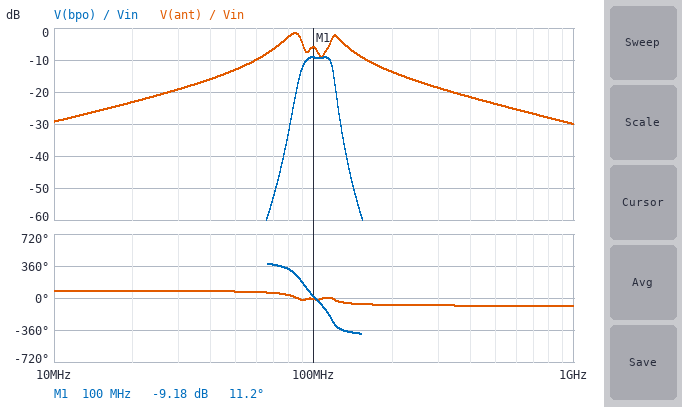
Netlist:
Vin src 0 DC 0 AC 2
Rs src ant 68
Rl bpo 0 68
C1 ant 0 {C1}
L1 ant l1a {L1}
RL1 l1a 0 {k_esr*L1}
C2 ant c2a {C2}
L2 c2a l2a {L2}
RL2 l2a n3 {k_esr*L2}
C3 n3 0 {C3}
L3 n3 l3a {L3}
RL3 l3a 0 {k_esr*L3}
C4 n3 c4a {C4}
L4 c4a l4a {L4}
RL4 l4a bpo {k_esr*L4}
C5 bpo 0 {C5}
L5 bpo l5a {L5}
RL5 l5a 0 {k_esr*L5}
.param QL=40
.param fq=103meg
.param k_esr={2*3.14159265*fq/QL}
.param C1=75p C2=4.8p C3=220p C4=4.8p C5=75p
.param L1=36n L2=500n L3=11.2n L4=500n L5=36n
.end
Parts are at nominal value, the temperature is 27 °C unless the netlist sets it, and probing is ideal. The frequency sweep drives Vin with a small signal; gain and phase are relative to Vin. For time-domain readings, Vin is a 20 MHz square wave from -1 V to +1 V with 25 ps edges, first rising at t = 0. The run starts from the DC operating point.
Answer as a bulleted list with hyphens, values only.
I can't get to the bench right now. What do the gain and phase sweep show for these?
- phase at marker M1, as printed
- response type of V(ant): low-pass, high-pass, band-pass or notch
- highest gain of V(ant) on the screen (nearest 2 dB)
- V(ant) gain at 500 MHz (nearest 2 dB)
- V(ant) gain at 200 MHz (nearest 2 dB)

- 11.2 deg
- band-pass
- -2 dB
- -24 dB
- -14 dB
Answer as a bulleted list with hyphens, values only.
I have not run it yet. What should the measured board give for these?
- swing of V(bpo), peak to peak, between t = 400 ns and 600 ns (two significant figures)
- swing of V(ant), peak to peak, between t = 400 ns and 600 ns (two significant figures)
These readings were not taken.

- 180 mV
- 890 mV
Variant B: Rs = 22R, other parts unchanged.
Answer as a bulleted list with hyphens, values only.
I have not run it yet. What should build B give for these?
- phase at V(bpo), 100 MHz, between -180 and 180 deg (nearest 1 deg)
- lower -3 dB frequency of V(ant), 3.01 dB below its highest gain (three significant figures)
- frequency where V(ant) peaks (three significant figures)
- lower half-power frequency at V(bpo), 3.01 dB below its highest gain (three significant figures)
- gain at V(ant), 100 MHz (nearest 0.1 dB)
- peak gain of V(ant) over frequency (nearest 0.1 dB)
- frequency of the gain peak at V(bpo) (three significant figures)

- 18 deg
- 57.3 MHz
- 83.6 MHz
- 91.6 MHz
- -2.4 dB
- -0.5 dB
- 107 MHz
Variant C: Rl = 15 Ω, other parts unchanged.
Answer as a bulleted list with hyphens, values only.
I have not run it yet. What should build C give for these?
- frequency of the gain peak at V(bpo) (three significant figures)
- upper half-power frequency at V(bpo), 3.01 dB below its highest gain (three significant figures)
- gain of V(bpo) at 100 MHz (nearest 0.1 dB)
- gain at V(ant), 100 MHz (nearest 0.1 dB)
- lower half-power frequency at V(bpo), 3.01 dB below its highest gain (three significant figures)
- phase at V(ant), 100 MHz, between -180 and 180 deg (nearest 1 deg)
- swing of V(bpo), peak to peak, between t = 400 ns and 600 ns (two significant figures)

- 107 MHz
- 115 MHz
- -17.9 dB
- -7.9 dB
- 91.9 MHz
- -30 deg
- 66 mV
